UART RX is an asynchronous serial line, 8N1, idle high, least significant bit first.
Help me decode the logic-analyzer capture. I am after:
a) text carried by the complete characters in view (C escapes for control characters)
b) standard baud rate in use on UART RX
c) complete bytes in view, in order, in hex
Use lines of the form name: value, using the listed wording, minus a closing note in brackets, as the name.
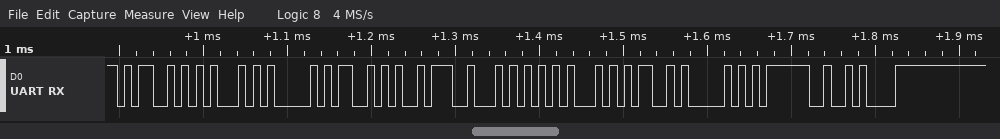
text carried by the complete characters in view: "MEAS:TEMP?\n"
standard baud rate in use on UART RX: 115200 baud
complete bytes in view, in order, in hex: 0x4D 0x45 0x41 0x53 0x3A 0x54 0x45 0x4D 0x50 0x3F 0x0A
